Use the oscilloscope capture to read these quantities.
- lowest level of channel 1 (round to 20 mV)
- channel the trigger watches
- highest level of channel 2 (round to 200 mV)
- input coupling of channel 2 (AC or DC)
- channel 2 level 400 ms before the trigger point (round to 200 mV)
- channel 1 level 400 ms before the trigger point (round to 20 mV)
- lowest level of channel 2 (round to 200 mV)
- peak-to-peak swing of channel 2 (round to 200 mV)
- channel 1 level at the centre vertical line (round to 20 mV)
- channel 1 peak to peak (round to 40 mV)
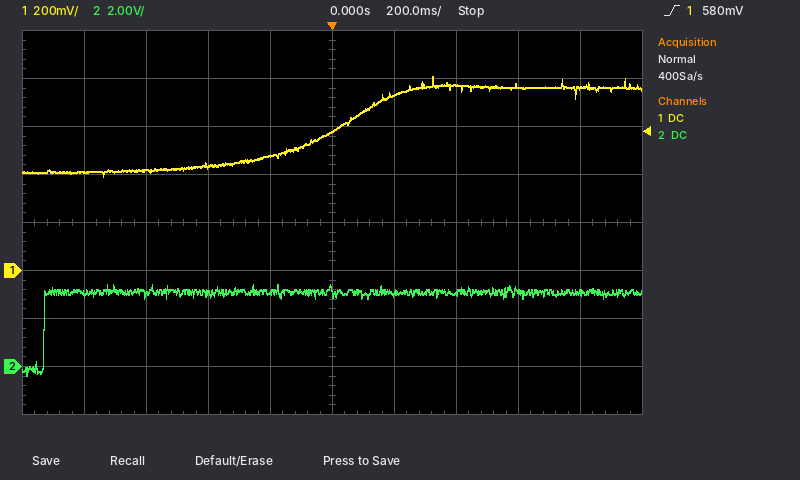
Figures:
400 mV
channel 1
3.4 V
DC
3.0 V
440 mV
-400 mV
3.8 V
580 mV
400 mV
